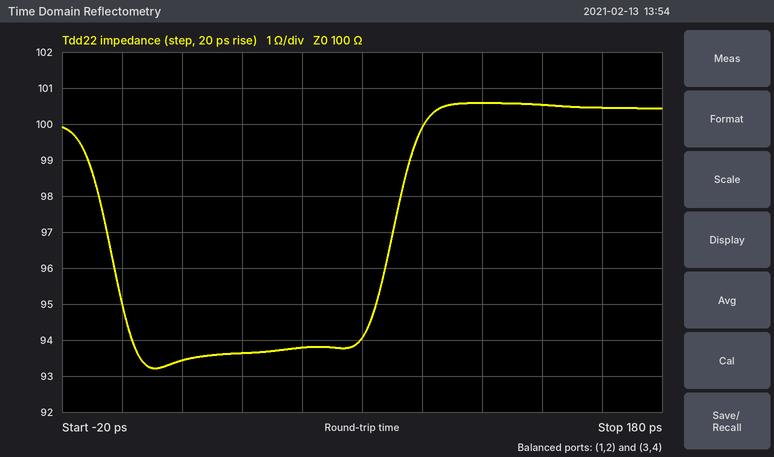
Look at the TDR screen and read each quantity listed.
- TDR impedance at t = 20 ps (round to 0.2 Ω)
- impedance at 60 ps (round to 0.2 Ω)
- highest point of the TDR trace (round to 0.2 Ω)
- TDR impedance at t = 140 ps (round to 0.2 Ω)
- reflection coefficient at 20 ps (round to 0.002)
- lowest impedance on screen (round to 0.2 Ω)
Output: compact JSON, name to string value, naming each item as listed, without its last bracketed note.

{"TDR impedance at t = 20 ps": "93.4 Ω", "impedance at 60 ps": "93.8 Ω", "highest point of the TDR trace": "100.6 Ω", "TDR impedance at t = 140 ps": "100.6 Ω", "reflection coefficient at 20 ps": "-0.034", "lowest impedance on screen": "93.2 Ω"}
